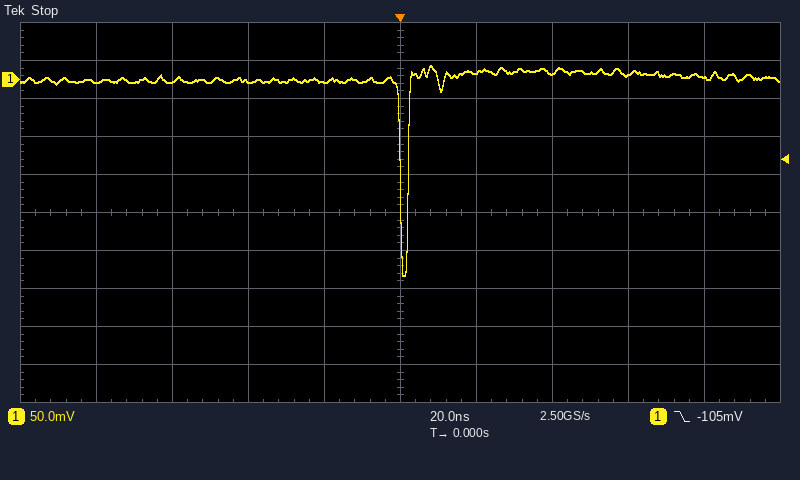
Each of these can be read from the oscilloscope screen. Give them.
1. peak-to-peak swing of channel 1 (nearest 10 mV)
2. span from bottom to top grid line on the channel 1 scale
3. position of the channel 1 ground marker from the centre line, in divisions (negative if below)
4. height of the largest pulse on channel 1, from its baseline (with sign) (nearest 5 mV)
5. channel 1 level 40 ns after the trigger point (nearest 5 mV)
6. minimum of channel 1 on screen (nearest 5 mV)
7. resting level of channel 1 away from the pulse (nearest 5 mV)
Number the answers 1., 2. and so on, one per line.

1. 280 mV
2. 500 mV
3. +3.5 div
4. -260 mV
5. 10 mV
6. -260 mV
7. 0 mV
